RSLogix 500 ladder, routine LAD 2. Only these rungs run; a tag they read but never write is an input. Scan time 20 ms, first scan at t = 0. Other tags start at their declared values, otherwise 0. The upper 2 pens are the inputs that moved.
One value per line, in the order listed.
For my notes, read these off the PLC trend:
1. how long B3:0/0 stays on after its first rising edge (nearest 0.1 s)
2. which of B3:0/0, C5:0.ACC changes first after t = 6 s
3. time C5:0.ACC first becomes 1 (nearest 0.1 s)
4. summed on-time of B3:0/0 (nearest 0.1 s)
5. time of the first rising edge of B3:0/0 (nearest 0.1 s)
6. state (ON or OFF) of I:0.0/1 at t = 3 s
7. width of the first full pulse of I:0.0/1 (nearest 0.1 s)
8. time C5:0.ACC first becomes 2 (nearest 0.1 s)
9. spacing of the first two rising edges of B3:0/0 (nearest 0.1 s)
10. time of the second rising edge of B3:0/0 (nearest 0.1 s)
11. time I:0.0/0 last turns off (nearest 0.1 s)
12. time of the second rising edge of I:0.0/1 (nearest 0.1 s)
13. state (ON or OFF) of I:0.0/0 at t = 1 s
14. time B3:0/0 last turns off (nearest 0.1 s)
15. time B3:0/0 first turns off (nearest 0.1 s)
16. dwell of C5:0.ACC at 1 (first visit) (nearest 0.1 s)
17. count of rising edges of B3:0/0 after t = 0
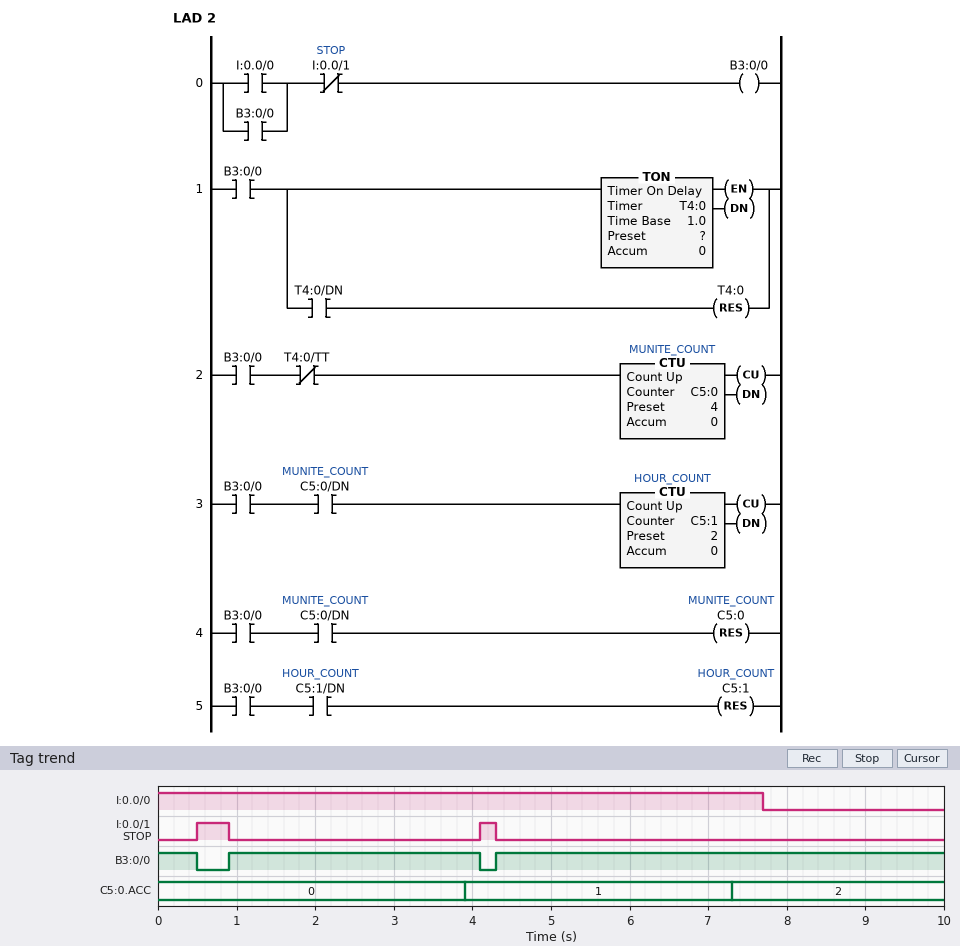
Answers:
3.2 s
C5:0.ACC
3.9 s
9.4 s
0.9 s
OFF
0.4 s
7.3 s
3.4 s
4.3 s
7.7 s
4.1 s
ON
4.1 s
0.5 s
3.4 s
2
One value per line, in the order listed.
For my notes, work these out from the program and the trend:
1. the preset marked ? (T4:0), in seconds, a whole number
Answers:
3 s
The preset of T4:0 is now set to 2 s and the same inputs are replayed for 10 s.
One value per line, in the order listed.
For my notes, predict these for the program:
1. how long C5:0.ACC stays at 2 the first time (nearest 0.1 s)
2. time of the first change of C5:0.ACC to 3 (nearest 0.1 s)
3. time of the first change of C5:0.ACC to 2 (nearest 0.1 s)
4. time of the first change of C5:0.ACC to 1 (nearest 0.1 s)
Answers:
2.0 s
8.3 s
6.3 s
2.9 s
